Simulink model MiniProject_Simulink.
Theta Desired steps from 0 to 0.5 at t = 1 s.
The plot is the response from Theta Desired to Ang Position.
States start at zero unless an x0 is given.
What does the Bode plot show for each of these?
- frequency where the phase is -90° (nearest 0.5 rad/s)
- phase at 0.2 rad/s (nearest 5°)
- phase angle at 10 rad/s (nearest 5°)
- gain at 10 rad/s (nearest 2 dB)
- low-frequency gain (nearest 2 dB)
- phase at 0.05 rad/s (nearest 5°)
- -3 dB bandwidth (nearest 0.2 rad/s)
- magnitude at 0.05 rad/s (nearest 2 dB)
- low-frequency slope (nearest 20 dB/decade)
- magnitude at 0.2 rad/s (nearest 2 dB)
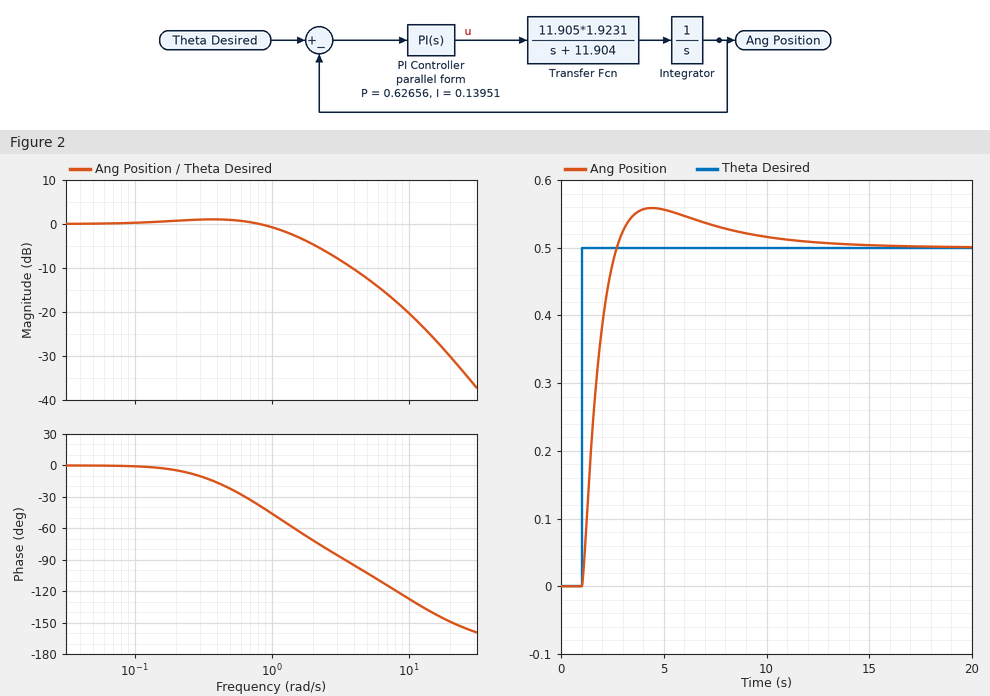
3.5 rad/s
-5°
-125°
-20 dB
0 dB
0°
1.6 rad/s
0 dB
0 dB/decade
0 dB
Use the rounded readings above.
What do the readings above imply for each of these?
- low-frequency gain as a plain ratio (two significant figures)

1.0
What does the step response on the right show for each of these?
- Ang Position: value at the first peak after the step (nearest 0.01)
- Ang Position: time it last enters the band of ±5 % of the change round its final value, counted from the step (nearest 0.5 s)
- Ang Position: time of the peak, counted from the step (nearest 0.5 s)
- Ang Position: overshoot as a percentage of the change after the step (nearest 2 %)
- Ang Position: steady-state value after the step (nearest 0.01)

0.56
7.5 s
3.5 s
12 %
0.50
